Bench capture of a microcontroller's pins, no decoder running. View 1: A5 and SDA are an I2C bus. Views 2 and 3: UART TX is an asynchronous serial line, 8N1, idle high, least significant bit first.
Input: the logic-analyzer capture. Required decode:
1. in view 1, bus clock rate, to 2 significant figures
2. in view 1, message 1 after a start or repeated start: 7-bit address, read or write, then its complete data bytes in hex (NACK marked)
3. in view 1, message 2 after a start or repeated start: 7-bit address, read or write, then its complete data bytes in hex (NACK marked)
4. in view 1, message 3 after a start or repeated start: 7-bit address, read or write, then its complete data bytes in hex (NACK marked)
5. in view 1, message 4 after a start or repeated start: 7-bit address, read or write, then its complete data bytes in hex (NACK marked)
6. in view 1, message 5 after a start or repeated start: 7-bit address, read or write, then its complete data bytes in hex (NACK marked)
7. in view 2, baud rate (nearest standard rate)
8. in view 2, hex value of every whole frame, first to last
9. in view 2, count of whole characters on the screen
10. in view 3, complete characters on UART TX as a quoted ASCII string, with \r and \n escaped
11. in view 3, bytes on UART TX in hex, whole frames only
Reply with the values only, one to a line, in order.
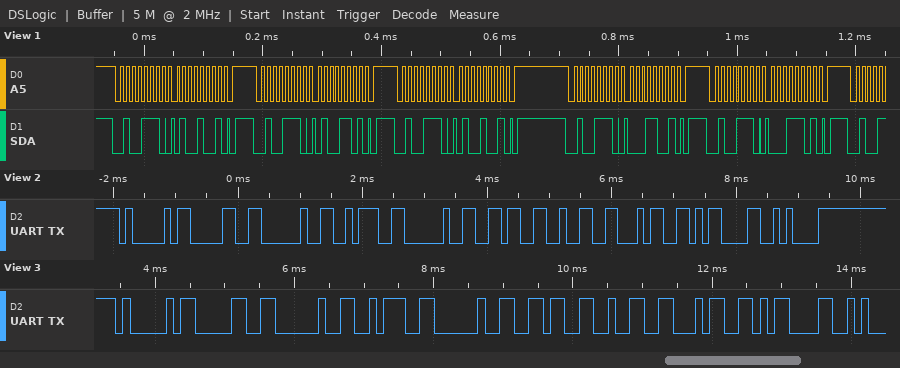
100 kHz
0x27 write: 49
0x27 write: 4D
0x27 write: 49
0x27 write: 19
0x27 write: 1D
9600 baud
41 30 20 3A 20 36 32 34 0D 0A
10
"A0 : 624\r"
0x41 0x30 0x20 0x3A 0x20 0x36 0x32 0x34 0x0D
